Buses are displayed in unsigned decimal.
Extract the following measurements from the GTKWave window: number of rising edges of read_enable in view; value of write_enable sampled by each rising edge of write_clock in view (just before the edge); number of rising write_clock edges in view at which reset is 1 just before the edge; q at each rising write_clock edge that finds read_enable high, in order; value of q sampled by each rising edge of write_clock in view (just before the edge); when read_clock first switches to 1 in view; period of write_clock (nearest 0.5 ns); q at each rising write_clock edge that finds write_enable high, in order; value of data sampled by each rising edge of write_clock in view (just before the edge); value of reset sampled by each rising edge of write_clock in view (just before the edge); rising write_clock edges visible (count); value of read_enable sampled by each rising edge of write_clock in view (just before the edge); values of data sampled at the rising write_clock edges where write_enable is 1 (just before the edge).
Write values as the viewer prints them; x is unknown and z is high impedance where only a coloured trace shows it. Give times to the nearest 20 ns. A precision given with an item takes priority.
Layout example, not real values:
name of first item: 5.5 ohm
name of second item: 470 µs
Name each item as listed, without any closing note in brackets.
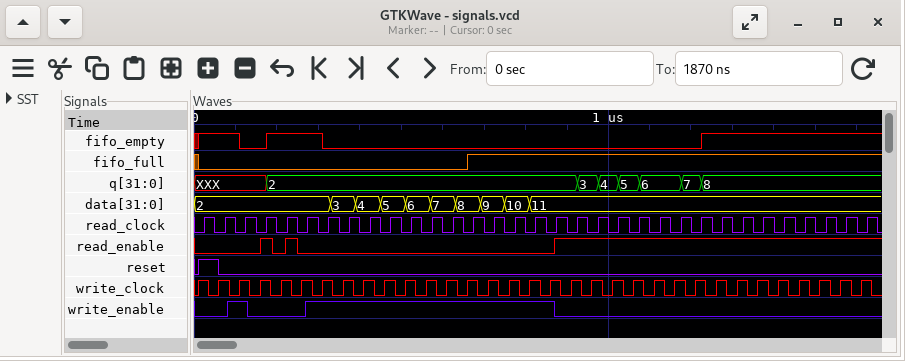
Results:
number of rising edges of read_enable in view: 3
value of write_enable sampled by each rising edge of write_clock in view: 0 0 1 0 0 0 1 1 1 1 1 1 1 1 1 1 1 1 0 0 0 0 0 0 0 0 0 0 0 0 0 0 0
number of rising write_clock edges in view at which reset is 1 just before the edge: 1
q at each rising write_clock edge that finds read_enable high, in order: 2, 3, 4, 5, 6, 6, 7, 8, 8, 8, 8, 8, 8, 8, 8
value of q sampled by each rising edge of write_clock in view: XXX, XXX, XXX, XXX, 2, 2, 2, 2, 2, 2, 2, 2, 2, 2, 2, 2, 2, 2, 2, 3, 4, 5, 6, 6, 7, 8, 8, 8, 8, 8, 8, 8, 8
when read_clock first switches to 1 in view: 20 ns
period of write_clock: 50 ns
q at each rising write_clock edge that finds write_enable high, in order: XXX, 2, 2, 2, 2, 2, 2, 2, 2, 2, 2, 2, 2
value of data sampled by each rising edge of write_clock in view: 2, 2, 2, 2, 2, 2, 2, 3, 4, 5, 5, 6, 7, 8, 9, 10, 10, 11, 11, 11, 11, 11, 11, 11, 11, 11, 11, 11, 11, 11, 11, 11, 11
value of reset sampled by each rising edge of write_clock in view: 0 1 0 0 0 0 0 0 0 0 0 0 0 0 0 0 0 0 0 0 0 0 0 0 0 0 0 0 0 0 0 0 0
rising write_clock edges visible: 33
value of read_enable sampled by each rising edge of write_clock in view: 0 0 0 0 0 0 0 0 0 0 0 0 0 0 0 0 0 0 1 1 1 1 1 1 1 1 1 1 1 1 1 1 1
values of data sampled at the rising write_clock edges where write_enable is 1: 2, 2, 3, 4, 5, 5, 6, 7, 8, 9, 10, 10, 11
